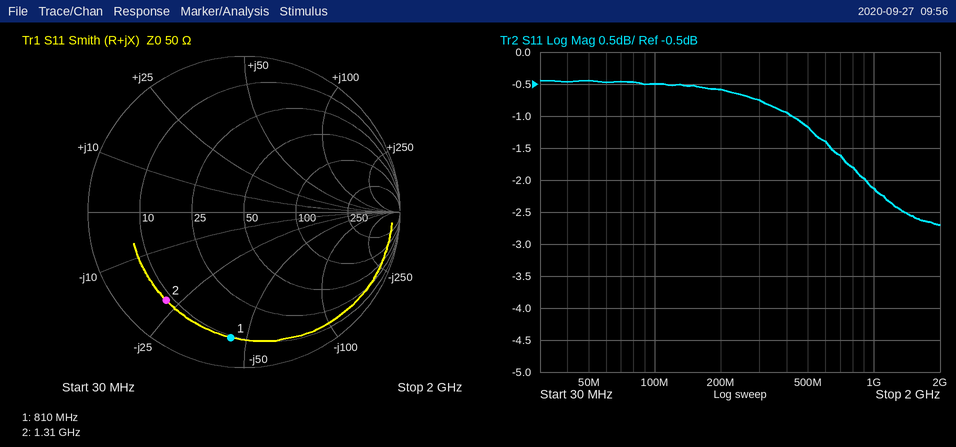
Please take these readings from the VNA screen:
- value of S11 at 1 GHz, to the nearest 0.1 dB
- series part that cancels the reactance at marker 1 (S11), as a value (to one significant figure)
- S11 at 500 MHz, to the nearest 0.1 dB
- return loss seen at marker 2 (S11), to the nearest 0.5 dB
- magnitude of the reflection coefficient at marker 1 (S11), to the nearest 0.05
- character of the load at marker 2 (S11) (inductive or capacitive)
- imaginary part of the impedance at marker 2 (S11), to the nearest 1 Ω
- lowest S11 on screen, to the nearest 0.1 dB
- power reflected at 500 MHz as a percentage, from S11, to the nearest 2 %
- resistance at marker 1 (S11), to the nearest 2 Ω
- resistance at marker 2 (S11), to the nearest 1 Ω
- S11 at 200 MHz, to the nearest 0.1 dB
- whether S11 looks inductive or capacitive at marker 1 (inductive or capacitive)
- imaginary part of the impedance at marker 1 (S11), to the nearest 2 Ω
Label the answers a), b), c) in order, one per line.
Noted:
a) -2.1 dB
b) 9 nH
c) -1.2 dB
d) 2.5 dB
e) 0.80
f) capacitive
g) -22 Ω
h) -2.7 dB
i) 76 %
j) 10 Ω
k) 8 Ω
l) -0.6 dB
m) capacitive
n) -44 Ω
